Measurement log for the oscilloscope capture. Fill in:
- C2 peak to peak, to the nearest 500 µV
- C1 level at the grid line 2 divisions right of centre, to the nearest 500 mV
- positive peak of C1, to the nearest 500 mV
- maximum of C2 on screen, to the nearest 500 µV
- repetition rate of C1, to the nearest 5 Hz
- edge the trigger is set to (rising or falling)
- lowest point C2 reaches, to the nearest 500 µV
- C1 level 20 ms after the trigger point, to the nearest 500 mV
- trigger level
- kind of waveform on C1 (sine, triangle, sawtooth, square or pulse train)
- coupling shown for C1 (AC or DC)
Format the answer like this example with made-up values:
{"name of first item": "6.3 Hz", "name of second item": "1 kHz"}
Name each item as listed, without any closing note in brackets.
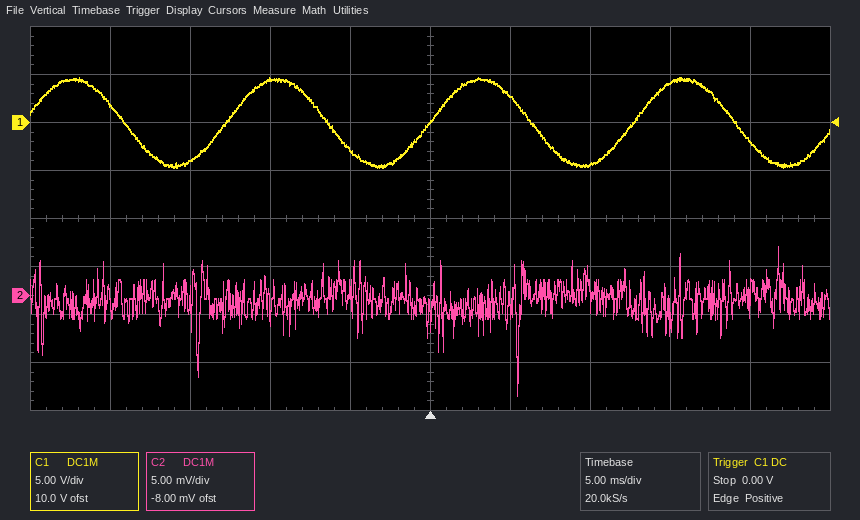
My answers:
{"C2 peak to peak, to the nearest 500 µV": "15.5 mV", "C1 level at the grid line 2 divisions right of centre, to the nearest 500 mV": "-4.5 V", "positive peak of C1, to the nearest 500 mV": "4.5 V", "maximum of C2 on screen, to the nearest 500 µV": "5.0 mV", "repetition rate of C1, to the nearest 5 Hz": "80 Hz", "edge the trigger is set to": "rising", "lowest point C2 reaches, to the nearest 500 µV": "-10.5 mV", "C1 level 20 ms after the trigger point, to the nearest 500 mV": "-2.0 V", "trigger level": "0.00 V", "kind of waveform on C1": "sine", "coupling shown for C1": "DC"}
